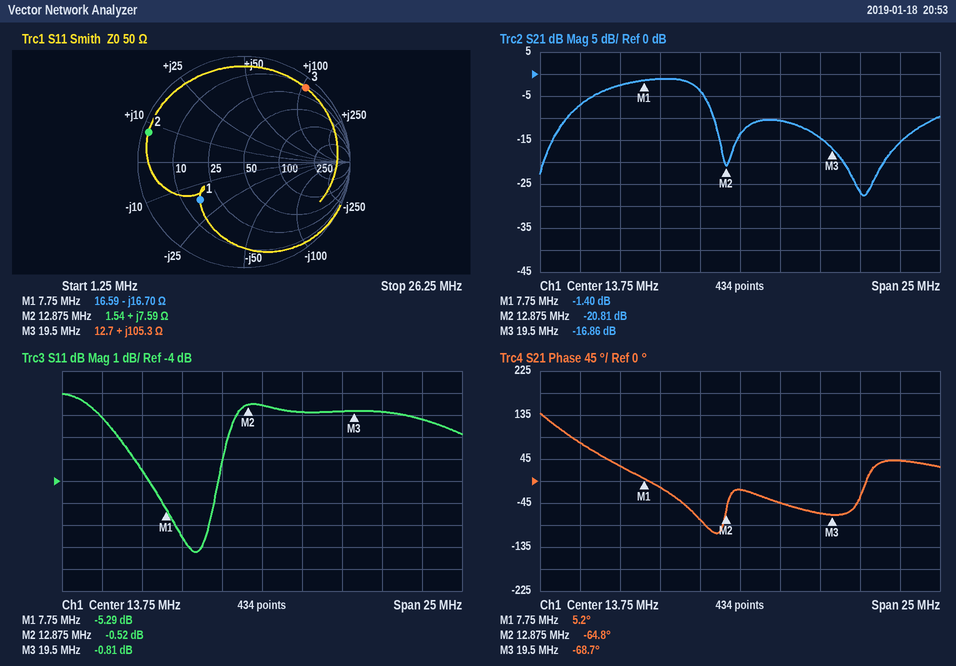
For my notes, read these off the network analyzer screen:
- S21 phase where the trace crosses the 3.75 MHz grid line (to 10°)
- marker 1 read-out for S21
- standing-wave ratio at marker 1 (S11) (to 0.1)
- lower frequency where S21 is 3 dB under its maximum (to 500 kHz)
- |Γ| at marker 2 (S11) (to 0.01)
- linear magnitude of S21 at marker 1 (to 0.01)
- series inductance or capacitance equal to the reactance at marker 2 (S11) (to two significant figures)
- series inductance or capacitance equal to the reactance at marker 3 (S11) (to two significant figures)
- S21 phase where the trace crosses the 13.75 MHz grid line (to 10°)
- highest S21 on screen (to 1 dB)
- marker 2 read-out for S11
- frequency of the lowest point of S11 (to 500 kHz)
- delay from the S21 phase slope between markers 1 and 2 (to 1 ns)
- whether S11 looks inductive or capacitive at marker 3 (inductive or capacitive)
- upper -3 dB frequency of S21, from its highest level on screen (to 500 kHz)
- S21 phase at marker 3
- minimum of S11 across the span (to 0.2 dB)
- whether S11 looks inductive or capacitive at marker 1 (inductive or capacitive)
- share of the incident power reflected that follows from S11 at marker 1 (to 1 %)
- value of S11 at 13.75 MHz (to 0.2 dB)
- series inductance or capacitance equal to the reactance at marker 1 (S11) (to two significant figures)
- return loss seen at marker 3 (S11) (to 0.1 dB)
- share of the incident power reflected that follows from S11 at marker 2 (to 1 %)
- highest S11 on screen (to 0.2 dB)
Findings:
80°
-1.40 dB
3.4
5.0 MHz
0.94
0.85
94 nH
860 nH
-20°
-1 dB
-0.52 dB
9.5 MHz
38 ns
inductive
11.5 MHz
-68.7°
-7.2 dB
capacitive
30 %
-0.6 dB
1.2 nF
0.8 dB
89 %
0.0 dB
